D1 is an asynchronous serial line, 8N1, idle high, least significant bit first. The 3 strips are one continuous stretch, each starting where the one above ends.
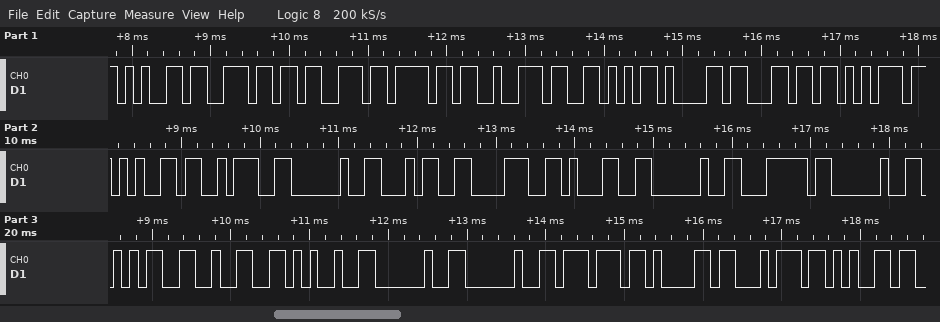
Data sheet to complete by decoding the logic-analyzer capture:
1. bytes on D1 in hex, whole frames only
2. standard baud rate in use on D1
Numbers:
65 6E 73 6F 72 56 61 6C 75 65 3A 20 34 38 31 20 7C 20 35 32 25 20 20 77 61 74 65
9600 baud
